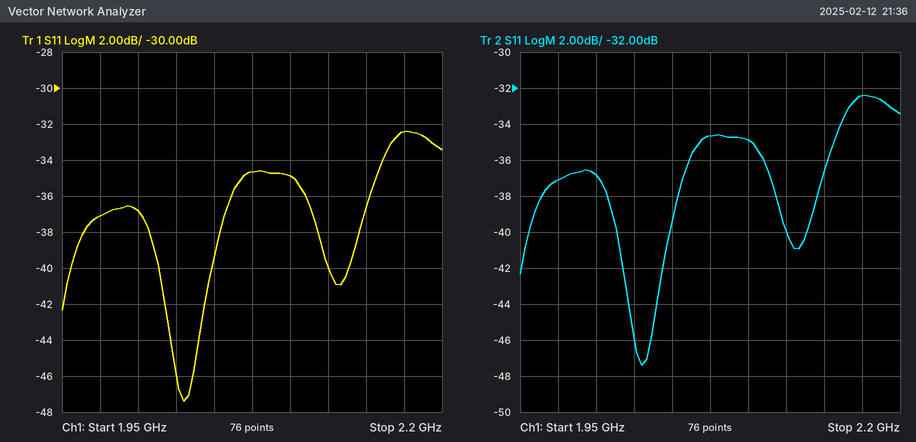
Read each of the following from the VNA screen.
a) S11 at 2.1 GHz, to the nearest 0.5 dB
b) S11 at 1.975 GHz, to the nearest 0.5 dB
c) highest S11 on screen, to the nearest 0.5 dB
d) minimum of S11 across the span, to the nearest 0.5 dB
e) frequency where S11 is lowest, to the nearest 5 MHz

-35.0 dB
-37.0 dB
-32.5 dB
-47.5 dB
2.030 GHz
